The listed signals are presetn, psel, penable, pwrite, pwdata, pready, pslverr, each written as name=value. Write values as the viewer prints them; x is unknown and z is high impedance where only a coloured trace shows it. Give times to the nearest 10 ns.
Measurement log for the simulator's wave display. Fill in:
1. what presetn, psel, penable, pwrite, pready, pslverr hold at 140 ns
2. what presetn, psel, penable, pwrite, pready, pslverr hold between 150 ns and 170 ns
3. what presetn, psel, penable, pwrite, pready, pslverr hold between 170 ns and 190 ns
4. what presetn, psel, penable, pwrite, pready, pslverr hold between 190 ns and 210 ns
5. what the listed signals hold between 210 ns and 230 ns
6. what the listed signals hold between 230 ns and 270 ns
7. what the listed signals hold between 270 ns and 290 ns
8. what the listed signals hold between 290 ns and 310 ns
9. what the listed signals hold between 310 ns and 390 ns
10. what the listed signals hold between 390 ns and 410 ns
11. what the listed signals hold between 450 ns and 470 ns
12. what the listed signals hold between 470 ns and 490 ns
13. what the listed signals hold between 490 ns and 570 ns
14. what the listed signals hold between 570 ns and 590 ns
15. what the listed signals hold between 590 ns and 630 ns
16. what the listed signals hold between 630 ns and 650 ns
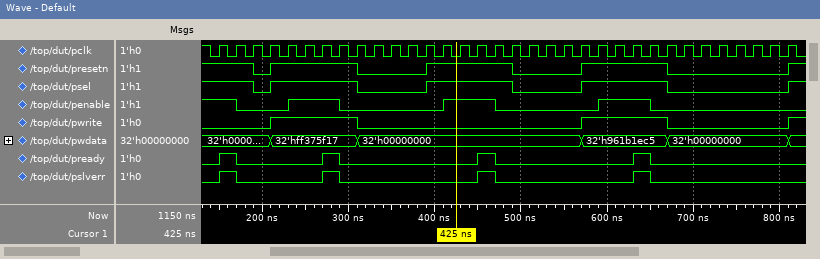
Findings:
presetn=1, psel=1, penable=1, pwrite=0, pready=0, pslverr=0
presetn=1, psel=1, penable=1, pwrite=0, pready=1, pslverr=1
presetn=1, psel=1, penable=0, pwrite=0, pready=0, pslverr=0
presetn=0, psel=0, penable=0, pwrite=0, pready=0, pslverr=0
presetn=1, psel=1, penable=0, pwrite=1, pwdata=32'hff375f17, pready=0, pslverr=0
presetn=1, psel=1, penable=1, pwrite=1, pwdata=32'hff375f17, pready=0, pslverr=0
presetn=1, psel=1, penable=1, pwrite=1, pwdata=32'hff375f17, pready=1, pslverr=1
presetn=1, psel=1, penable=0, pwrite=1, pwdata=32'hff375f17, pready=0, pslverr=0
presetn=0, psel=0, penable=0, pwrite=0, pwdata=32'h00000000, pready=0, pslverr=0
presetn=1, psel=1, penable=0, pwrite=0, pwdata=32'h00000000, pready=0, pslverr=0
presetn=1, psel=1, penable=1, pwrite=0, pwdata=32'h00000000, pready=1, pslverr=1
presetn=1, psel=1, penable=0, pwrite=0, pwdata=32'h00000000, pready=0, pslverr=0
presetn=0, psel=0, penable=0, pwrite=0, pwdata=32'h00000000, pready=0, pslverr=0
presetn=1, psel=1, penable=0, pwrite=1, pwdata=32'h961b1ec5, pready=0, pslverr=0
presetn=1, psel=1, penable=1, pwrite=1, pwdata=32'h961b1ec5, pready=0, pslverr=0
presetn=1, psel=1, penable=1, pwrite=1, pwdata=32'h961b1ec5, pready=1, pslverr=1
